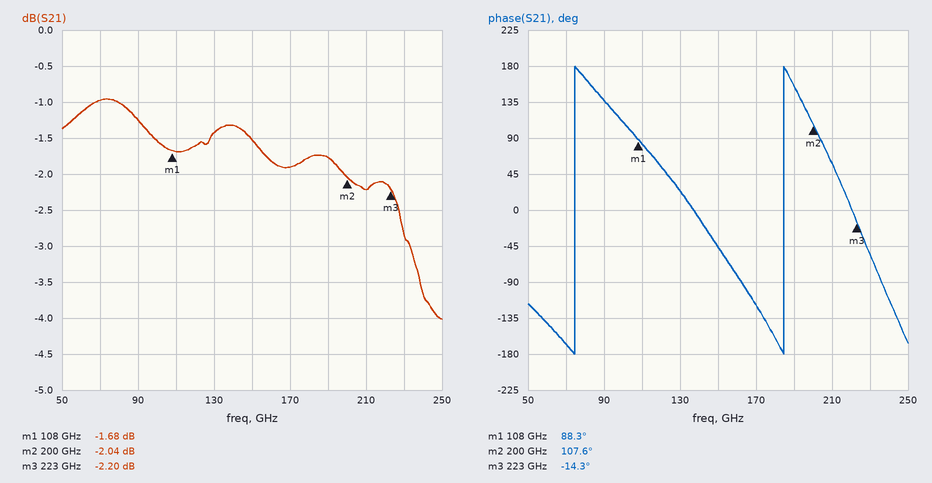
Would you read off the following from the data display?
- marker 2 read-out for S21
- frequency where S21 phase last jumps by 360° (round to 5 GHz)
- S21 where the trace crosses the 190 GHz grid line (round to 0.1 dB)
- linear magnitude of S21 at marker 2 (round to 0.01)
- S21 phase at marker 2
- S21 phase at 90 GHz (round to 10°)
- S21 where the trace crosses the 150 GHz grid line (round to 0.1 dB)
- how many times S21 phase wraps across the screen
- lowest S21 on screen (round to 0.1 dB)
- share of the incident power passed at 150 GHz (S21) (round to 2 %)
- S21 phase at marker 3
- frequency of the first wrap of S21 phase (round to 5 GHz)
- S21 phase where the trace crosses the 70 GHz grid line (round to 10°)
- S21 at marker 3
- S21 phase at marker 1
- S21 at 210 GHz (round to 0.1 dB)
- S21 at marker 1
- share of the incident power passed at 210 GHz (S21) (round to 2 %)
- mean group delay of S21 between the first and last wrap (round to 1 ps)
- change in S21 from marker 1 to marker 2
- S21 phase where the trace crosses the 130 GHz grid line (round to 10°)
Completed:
-2.04 dB
185 GHz
-1.8 dB
0.79
107.6°
140°
-1.5 dB
2
-4.0 dB
70 %
-14.3°
75 GHz
-170°
-2.20 dB
88.3°
-2.2 dB
-1.68 dB
60 %
9 ps
-0.36 dB
20°
